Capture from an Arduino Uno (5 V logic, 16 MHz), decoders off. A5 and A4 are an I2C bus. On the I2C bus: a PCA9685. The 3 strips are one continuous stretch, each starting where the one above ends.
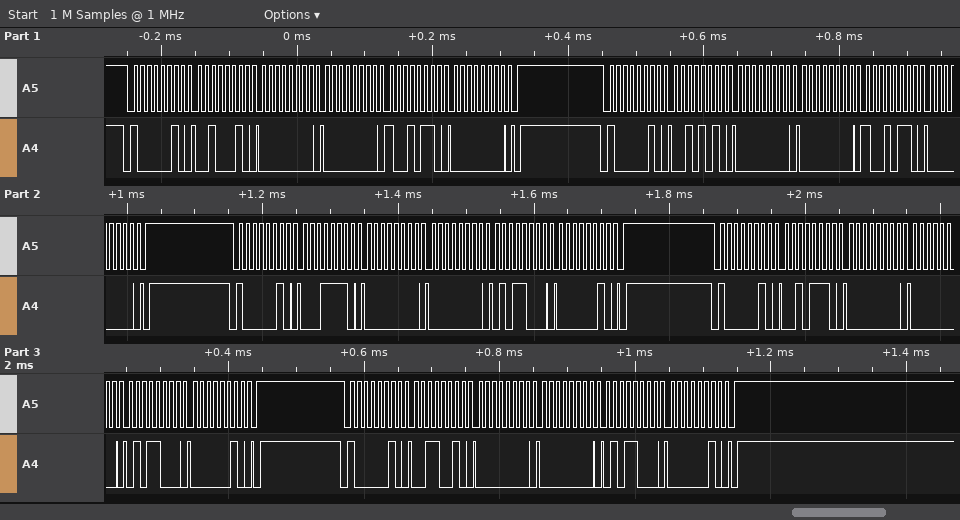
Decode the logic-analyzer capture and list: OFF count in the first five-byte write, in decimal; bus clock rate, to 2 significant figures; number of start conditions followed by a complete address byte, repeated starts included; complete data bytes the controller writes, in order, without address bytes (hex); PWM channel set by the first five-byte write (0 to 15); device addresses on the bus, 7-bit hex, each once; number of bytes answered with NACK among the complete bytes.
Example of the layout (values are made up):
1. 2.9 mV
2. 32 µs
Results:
1. 150
2. 100 kHz
3. 5
4. 22 00 00 96 00 2A 00 00 96 00 1E 00 00 58 02 2E 00 00 58 02 32 00 00 58 02
5. 7
6. 0x41
7. 0
